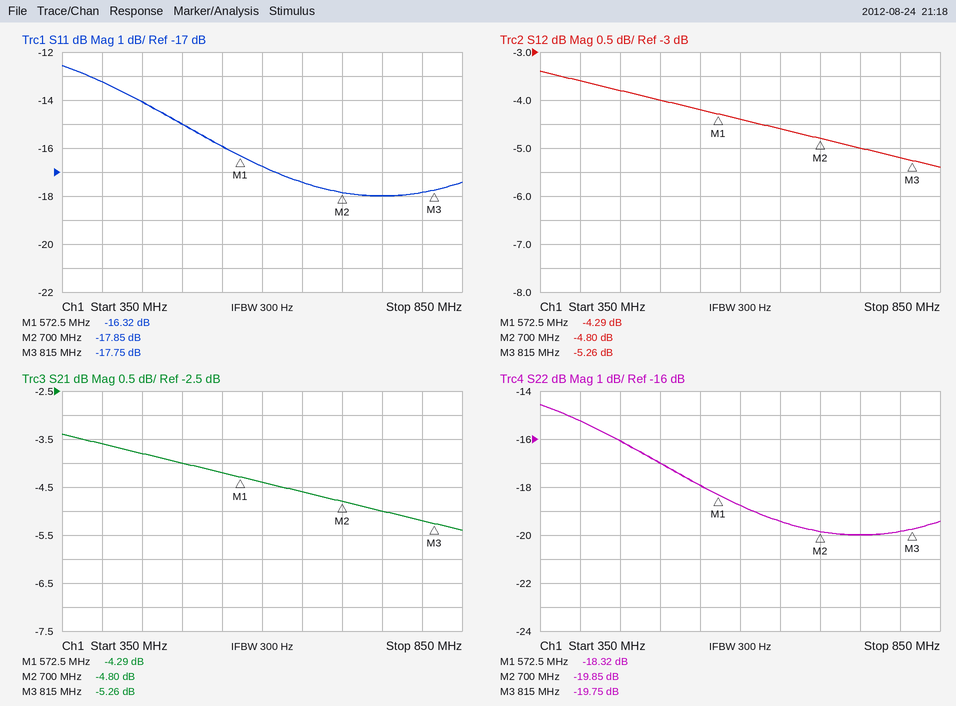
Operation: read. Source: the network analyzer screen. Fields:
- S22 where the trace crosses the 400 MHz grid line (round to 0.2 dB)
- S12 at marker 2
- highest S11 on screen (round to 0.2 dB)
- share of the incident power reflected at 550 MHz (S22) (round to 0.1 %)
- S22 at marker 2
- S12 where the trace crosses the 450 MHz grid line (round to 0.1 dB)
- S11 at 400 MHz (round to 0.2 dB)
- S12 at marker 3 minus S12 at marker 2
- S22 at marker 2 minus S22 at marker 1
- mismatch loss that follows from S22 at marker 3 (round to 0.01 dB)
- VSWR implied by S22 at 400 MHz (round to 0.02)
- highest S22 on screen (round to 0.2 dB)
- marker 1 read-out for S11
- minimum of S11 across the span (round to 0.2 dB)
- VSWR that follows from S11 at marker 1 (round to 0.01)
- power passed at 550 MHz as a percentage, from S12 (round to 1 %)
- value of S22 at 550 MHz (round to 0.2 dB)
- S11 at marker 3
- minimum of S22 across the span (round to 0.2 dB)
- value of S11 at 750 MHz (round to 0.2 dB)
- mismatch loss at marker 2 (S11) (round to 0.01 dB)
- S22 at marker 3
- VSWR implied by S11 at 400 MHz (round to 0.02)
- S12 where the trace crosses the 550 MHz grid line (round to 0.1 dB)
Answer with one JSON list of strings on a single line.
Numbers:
["-15.2 dB", "-4.80 dB", "-12.6 dB", "1.6 %", "-19.85 dB", "-3.8 dB", "-13.2 dB", "-0.46 dB", "-1.53 dB", "0.05 dB", "1.42", "-14.6 dB", "-16.32 dB", "-18.0 dB", "1.36", "38 %", "-18.0 dB", "-17.75 dB", "-20.0 dB", "-18.0 dB", "0.07 dB", "-19.75 dB", "1.56", "-4.2 dB"]
